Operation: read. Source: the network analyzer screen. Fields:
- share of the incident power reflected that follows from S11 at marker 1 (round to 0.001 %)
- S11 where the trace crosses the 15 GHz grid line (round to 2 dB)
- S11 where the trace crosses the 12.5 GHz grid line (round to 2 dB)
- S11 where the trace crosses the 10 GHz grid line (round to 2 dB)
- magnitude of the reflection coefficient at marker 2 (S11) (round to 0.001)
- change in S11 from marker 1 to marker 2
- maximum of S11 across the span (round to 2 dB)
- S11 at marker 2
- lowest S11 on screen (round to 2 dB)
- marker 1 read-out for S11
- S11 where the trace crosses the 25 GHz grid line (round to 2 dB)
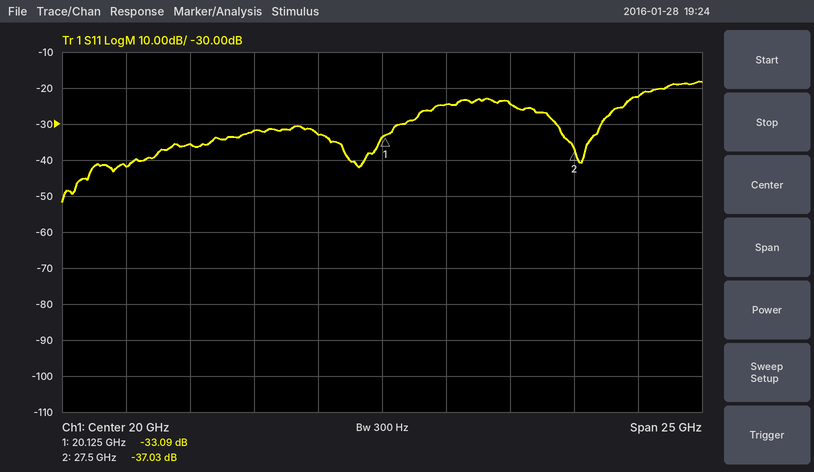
0.049 %
-32 dB
-36 dB
-42 dB
0.014
-3.94 dB
-18 dB
-37.03 dB
-52 dB
-33.09 dB
-24 dB
